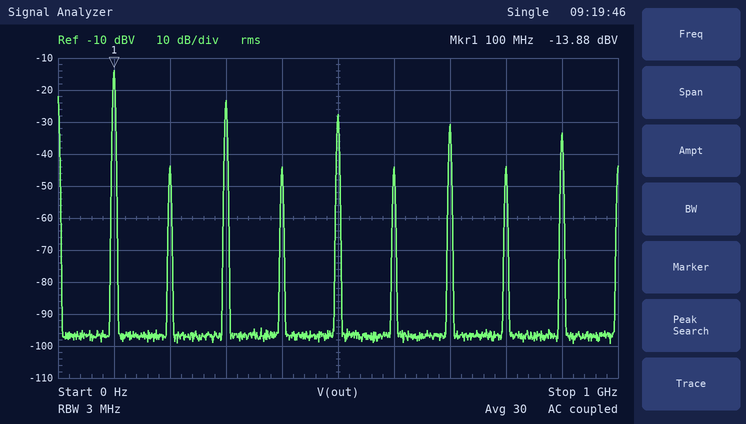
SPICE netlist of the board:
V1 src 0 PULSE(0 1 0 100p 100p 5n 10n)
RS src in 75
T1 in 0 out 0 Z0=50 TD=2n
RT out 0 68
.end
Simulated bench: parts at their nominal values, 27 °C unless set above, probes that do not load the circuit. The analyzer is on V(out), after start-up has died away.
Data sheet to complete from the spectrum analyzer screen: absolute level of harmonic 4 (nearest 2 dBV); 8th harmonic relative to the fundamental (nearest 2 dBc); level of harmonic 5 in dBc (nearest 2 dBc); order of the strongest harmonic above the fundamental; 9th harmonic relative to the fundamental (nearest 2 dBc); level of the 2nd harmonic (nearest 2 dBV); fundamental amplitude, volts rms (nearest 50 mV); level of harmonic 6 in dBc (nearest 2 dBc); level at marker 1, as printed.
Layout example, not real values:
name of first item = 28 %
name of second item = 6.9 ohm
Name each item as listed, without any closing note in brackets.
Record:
absolute level of harmonic 4 = -44 dBV
8th harmonic relative to the fundamental = -30 dBc
level of harmonic 5 in dBc = -14 dBc
order of the strongest harmonic above the fundamental = 3
9th harmonic relative to the fundamental = -20 dBc
level of the 2nd harmonic = -44 dBV
fundamental amplitude, volts rms = 200 mV
level of harmonic 6 in dBc = -30 dBc
level at marker 1, as printed = -13.88 dBV
